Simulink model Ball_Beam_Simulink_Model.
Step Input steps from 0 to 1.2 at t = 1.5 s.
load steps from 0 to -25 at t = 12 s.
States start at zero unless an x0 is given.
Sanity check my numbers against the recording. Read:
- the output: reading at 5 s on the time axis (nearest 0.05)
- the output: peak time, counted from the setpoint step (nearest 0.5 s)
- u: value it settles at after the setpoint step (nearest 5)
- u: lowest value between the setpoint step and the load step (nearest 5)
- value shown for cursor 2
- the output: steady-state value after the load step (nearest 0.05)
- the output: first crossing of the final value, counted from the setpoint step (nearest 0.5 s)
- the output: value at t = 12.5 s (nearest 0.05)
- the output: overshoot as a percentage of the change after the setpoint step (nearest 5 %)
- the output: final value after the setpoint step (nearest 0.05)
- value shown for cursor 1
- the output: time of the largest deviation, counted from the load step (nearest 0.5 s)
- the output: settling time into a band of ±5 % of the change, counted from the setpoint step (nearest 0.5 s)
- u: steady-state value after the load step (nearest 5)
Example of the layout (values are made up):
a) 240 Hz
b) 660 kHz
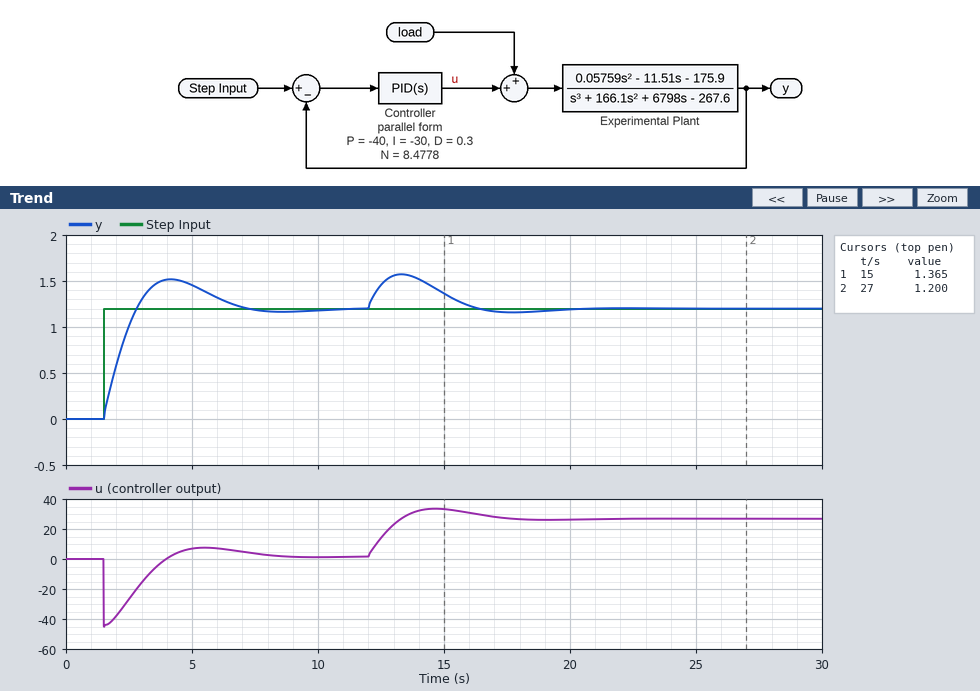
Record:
a) 1.45
b) 2.5 s
c) 0
d) -45
e) 1.200
f) 1.20
g) 1.5 s
h) 1.45
i) 25 %
j) 1.20
k) 1.365
l) 1.5 s
m) 5.0 s
n) 25
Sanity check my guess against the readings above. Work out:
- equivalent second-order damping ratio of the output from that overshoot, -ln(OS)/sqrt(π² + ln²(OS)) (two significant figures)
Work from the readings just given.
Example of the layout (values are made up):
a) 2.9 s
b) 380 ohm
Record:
a) 0.40
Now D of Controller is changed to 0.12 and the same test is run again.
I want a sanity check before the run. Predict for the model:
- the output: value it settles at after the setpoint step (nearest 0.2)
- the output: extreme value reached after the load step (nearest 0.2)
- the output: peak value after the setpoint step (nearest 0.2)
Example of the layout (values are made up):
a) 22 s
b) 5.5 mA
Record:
a) 1.2
b) 1.6
c) 1.6
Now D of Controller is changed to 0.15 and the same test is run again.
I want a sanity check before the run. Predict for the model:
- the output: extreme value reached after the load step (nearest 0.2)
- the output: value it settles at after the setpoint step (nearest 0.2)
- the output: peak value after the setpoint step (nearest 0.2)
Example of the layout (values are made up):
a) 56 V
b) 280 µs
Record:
a) 1.6
b) 1.2
c) 1.6
